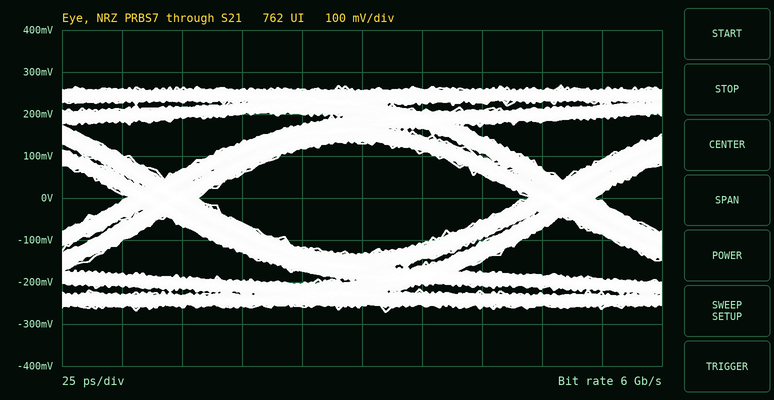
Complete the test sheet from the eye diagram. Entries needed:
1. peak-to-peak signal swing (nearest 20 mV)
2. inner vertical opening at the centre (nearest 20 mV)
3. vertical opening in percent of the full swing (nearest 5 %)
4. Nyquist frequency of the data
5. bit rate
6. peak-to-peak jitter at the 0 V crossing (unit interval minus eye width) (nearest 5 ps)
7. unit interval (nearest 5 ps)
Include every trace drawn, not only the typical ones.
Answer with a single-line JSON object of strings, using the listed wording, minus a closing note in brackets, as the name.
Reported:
{"peak-to-peak signal swing": "540 mV", "inner vertical opening at the centre": "260 mV", "vertical opening in percent of the full swing": "50 %", "Nyquist frequency of the data": "3 GHz", "bit rate": "6 Gb/s", "peak-to-peak jitter at the 0 V crossing (unit interval minus eye width)": "30 ps", "unit interval": "165 ps"}
